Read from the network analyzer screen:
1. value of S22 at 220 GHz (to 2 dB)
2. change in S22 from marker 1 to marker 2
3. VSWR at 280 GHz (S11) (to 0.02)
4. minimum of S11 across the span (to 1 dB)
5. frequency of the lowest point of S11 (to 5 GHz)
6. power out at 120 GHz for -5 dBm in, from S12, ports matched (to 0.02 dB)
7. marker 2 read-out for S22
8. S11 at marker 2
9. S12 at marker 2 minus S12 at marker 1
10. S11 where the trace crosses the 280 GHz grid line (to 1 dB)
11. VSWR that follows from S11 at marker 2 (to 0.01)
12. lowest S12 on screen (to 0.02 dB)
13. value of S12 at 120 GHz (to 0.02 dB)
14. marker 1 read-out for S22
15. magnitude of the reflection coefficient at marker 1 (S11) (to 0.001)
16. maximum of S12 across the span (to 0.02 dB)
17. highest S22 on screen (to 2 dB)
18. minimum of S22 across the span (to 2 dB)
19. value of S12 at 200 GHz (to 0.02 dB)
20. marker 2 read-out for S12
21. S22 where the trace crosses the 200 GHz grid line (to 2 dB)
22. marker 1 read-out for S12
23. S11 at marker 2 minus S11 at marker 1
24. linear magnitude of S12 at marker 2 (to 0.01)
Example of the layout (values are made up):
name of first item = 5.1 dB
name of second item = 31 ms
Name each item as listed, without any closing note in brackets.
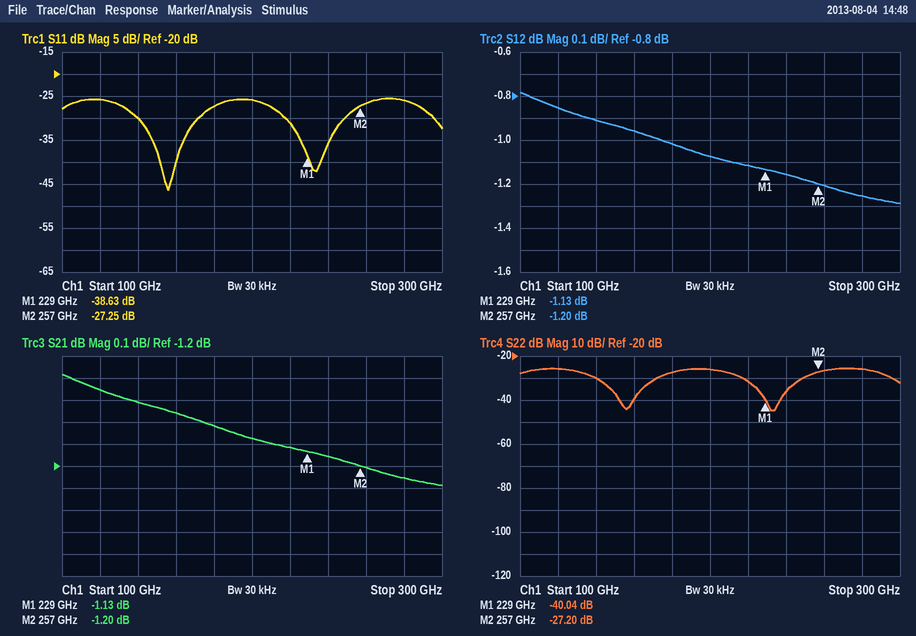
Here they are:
value of S22 at 220 GHz = -32 dB
change in S22 from marker 1 to marker 2 = 12.84 dB
VSWR at 280 GHz (S11) = 1.10
minimum of S11 across the span = -46 dB
frequency of the lowest point of S11 = 155 GHz
power out at 120 GHz for -5 dBm in, from S12, ports matched = -5.86 dBm
marker 2 read-out for S22 = -27.20 dB
S11 at marker 2 = -27.25 dB
S12 at marker 2 minus S12 at marker 1 = -0.07 dB
S11 where the trace crosses the 280 GHz grid line = -26 dB
VSWR that follows from S11 at marker 2 = 1.09
lowest S12 on screen = -1.28 dB
value of S12 at 120 GHz = -0.86 dB
marker 1 read-out for S22 = -40.04 dB
magnitude of the reflection coefficient at marker 1 (S11) = 0.012
maximum of S12 across the span = -0.78 dB
highest S22 on screen = -26 dB
minimum of S22 across the span = -44 dB
value of S12 at 200 GHz = -1.08 dB
marker 2 read-out for S12 = -1.20 dB
S22 where the trace crosses the 200 GHz grid line = -26 dB
marker 1 read-out for S12 = -1.13 dB
S11 at marker 2 minus S11 at marker 1 = 11.38 dB
linear magnitude of S12 at marker 2 = 0.87
